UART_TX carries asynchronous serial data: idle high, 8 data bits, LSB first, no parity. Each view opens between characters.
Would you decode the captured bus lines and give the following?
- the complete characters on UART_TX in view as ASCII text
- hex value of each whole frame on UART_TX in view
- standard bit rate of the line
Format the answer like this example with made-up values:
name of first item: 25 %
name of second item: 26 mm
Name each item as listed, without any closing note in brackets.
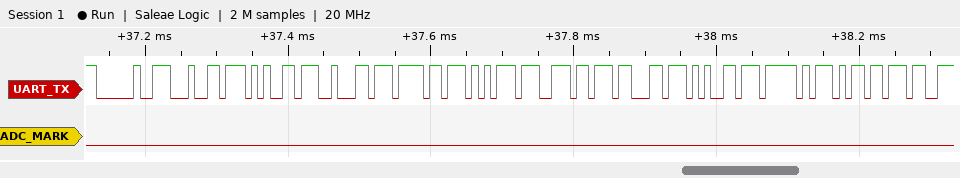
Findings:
the complete characters on UART_TX in view as ASCII text: " debounce_m"
hex value of each whole frame on UART_TX in view: 20, 64, 65, 62, 6F, 75, 6E, 63, 65, 5F, 6D
standard bit rate of the line: 115200 baud
